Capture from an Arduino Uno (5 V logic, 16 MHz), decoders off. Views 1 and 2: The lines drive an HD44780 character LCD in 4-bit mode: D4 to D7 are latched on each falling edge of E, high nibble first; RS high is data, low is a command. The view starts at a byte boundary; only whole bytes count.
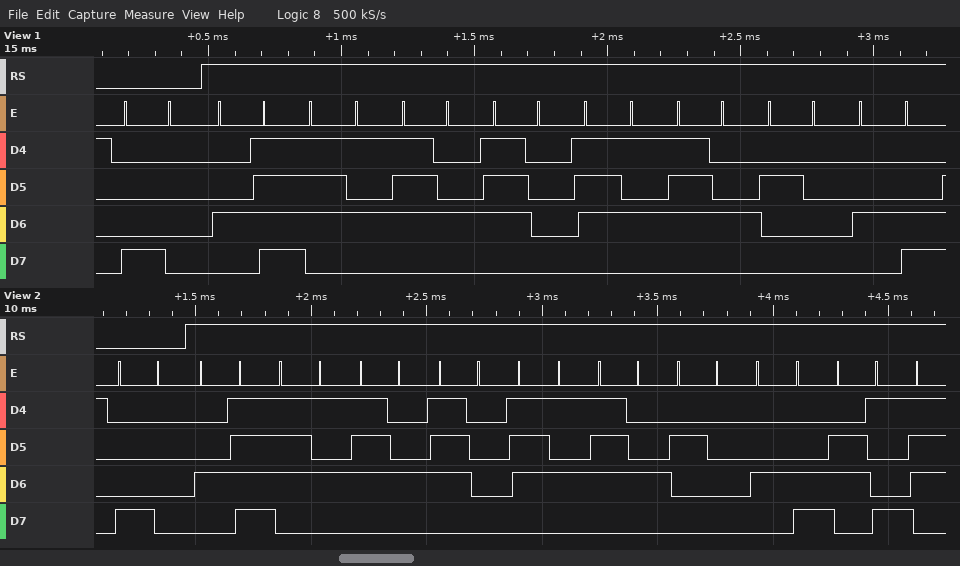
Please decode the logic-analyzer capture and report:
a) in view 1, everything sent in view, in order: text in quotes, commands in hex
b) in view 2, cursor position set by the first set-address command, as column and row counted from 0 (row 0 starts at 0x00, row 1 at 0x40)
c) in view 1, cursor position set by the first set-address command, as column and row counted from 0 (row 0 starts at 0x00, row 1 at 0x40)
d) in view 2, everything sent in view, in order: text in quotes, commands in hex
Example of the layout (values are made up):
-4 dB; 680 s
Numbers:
0x80 "Output L"; column 0, row 0; column 0, row 0; 0x80 "Output Li"
